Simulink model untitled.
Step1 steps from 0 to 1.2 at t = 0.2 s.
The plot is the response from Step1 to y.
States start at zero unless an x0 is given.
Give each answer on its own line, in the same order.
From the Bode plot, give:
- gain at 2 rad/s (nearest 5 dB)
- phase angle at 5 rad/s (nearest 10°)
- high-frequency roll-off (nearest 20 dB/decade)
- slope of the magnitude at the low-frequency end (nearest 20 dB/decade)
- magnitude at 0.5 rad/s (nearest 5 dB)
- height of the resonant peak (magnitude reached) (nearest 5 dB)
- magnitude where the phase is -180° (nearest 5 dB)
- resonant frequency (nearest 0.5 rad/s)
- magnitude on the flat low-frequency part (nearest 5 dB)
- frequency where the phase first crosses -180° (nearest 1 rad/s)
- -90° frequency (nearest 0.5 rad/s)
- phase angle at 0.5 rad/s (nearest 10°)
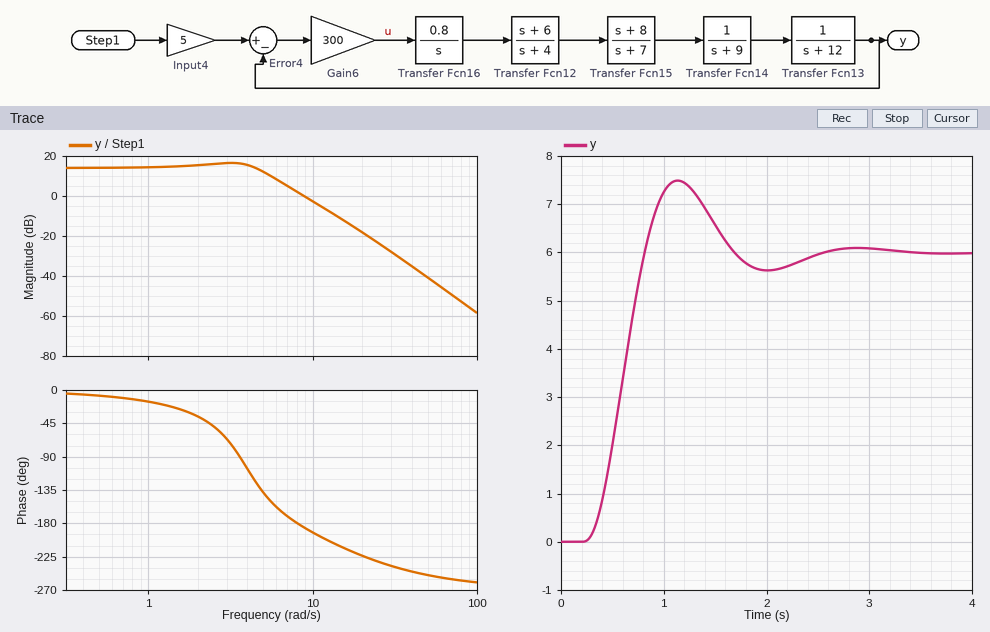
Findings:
15 dB
-140°
-60 dB/decade
0 dB/decade
15 dB
15 dB
0 dB
3.0 rad/s
15 dB
8 rad/s
3.5 rad/s
-10°
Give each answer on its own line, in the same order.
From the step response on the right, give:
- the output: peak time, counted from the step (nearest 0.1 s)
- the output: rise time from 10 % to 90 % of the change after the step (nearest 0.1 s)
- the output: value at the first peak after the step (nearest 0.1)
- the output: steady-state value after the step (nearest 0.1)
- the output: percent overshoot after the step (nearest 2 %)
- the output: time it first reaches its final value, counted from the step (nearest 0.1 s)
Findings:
0.9 s
0.4 s
7.5
6.0
24 %
0.6 s
